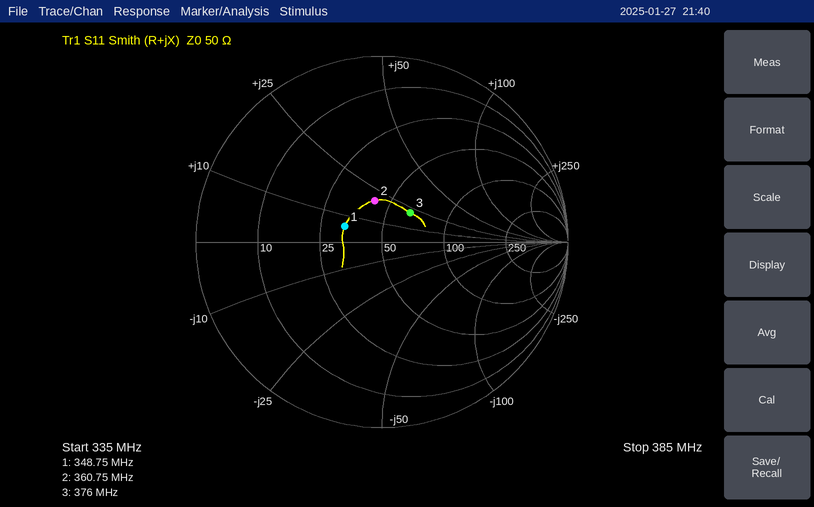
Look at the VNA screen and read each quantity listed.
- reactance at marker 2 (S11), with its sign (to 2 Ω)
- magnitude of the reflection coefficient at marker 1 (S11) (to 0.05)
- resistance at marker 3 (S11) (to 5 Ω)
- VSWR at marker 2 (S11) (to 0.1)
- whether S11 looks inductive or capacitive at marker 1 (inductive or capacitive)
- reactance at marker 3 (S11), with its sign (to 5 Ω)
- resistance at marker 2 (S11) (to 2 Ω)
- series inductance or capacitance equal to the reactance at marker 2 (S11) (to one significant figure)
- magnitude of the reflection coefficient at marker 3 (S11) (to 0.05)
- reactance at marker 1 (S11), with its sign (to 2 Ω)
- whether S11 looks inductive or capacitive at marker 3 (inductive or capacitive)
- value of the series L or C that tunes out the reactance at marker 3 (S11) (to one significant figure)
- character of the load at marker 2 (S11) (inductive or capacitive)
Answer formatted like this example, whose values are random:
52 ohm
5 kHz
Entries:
+20 Ω
0.20
65 Ω
1.6
inductive
+20 Ω
42 Ω
9 nH
0.20
+6 Ω
inductive
20 pF
inductive
